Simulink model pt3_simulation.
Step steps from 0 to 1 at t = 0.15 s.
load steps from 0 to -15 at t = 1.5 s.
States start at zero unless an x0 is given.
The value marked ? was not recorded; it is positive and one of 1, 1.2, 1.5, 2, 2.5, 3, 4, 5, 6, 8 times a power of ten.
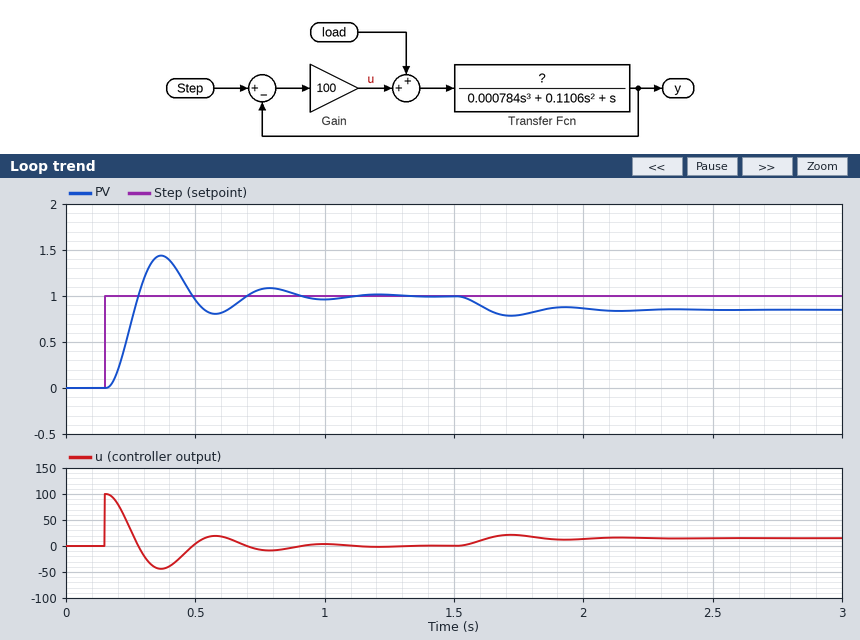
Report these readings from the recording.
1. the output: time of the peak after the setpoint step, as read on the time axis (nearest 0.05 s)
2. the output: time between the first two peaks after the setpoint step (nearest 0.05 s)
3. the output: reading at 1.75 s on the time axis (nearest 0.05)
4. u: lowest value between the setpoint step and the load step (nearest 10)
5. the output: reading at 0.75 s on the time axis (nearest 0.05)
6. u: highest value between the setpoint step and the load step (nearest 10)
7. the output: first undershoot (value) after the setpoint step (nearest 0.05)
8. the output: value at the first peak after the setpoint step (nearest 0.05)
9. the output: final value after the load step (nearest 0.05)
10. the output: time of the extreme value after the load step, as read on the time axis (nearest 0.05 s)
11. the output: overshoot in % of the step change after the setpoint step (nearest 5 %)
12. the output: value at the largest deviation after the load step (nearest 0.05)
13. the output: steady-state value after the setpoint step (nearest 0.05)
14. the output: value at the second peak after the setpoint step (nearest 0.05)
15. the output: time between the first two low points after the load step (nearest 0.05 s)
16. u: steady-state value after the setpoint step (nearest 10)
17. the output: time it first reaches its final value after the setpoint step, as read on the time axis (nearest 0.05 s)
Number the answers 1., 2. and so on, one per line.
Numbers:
1. 0.35 s
2. 0.40 s
3. 0.80
4. -40
5. 1.05
6. 100
7. 0.80
8. 1.45
9. 0.85
10. 1.70 s
11. 45 %
12. 0.80
13. 1.00
14. 1.10
15. 0.40 s
16. 0
17. 0.30 s
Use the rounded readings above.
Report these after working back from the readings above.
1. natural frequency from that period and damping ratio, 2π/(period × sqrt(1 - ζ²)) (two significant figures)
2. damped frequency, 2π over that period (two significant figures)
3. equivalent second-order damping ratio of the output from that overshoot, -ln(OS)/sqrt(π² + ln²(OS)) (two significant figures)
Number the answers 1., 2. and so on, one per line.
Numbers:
1. 16 rad/s
2. 16 rad/s
3. 0.25
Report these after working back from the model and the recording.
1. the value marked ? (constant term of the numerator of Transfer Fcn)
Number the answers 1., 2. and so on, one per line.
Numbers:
1. 0.25
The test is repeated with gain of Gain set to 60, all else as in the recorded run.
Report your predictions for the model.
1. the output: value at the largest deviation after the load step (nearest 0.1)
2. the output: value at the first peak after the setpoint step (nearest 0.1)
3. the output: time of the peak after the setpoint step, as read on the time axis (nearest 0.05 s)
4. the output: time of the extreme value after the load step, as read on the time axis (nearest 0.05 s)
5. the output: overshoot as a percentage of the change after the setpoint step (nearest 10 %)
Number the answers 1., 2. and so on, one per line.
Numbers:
1. 0.7
2. 1.3
3. 0.45 s
4. 1.80 s
5. 30 %
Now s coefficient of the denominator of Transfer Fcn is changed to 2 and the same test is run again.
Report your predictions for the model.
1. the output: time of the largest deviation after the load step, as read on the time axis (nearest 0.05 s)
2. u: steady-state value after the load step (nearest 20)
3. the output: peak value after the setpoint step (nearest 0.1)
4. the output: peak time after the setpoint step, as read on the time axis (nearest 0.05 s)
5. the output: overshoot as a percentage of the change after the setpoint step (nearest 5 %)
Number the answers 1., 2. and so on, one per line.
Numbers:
1. 1.75 s
2. 20
3. 1.1
4. 0.40 s
5. 10 %
